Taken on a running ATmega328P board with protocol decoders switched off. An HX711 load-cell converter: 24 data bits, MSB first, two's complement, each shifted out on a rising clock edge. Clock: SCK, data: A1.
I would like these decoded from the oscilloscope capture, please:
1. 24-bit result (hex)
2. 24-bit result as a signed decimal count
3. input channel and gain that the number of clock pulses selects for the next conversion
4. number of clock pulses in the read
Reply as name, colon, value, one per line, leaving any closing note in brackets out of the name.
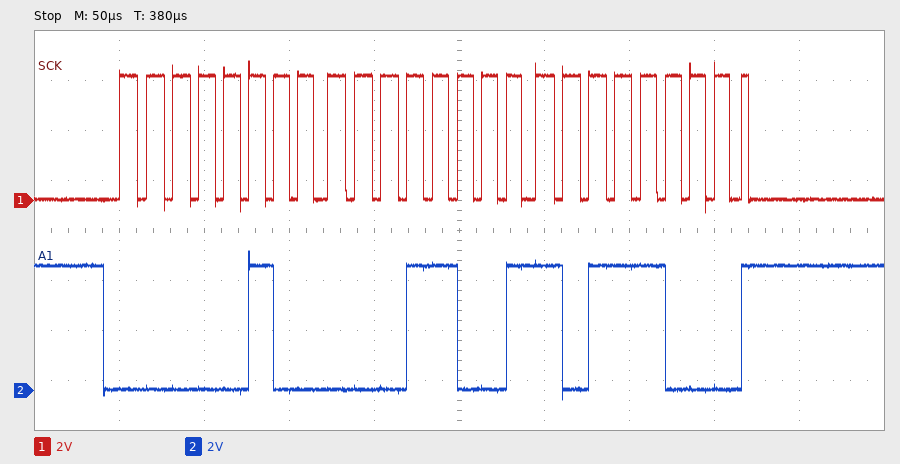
24-bit result: 0x0419B8
24-bit result as a signed decimal count: 268728
input channel and gain that the number of clock pulses selects for the next conversion: channel A, gain 128
number of clock pulses in the read: 25
